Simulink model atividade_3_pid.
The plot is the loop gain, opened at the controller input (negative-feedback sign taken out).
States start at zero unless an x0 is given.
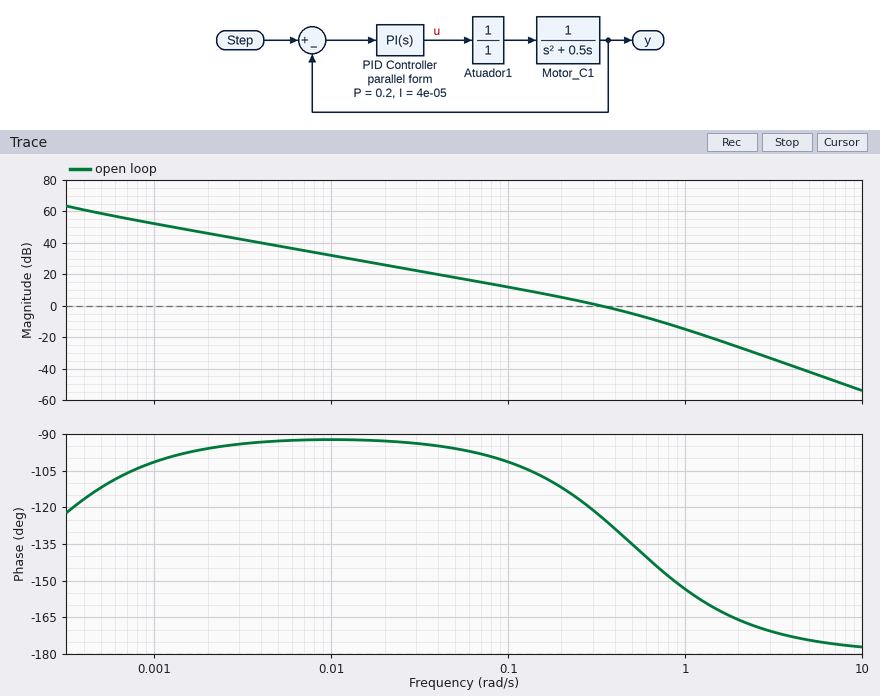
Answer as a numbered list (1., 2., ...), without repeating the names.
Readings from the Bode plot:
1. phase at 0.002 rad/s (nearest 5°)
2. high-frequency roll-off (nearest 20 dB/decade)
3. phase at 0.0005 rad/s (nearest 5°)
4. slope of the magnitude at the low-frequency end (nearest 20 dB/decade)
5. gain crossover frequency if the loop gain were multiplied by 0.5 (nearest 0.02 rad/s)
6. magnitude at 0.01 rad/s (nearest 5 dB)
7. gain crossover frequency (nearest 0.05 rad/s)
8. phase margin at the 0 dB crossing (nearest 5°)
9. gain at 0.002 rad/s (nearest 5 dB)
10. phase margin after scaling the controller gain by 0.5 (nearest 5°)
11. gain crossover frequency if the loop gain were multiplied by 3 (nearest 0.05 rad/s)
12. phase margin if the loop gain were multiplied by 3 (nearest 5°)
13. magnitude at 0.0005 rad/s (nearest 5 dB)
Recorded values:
1. -95°
2. -40 dB/decade
3. -110°
4. -20 dB/decade
5. 0.18 rad/s
6. 30 dB
7. 0.35 rad/s
8. 55°
9. 45 dB
10. 70°
11. 0.70 rad/s
12. 35°
13. 60 dB
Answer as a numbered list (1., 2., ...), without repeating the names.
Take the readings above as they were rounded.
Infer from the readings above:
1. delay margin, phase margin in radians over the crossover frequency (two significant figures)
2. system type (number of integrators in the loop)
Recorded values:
1. 2.7 s
2. 1
